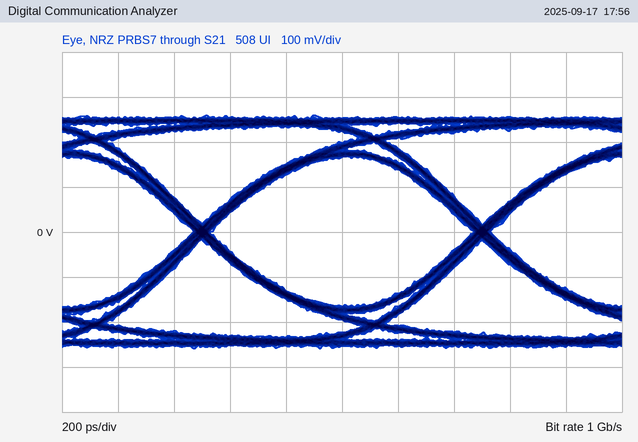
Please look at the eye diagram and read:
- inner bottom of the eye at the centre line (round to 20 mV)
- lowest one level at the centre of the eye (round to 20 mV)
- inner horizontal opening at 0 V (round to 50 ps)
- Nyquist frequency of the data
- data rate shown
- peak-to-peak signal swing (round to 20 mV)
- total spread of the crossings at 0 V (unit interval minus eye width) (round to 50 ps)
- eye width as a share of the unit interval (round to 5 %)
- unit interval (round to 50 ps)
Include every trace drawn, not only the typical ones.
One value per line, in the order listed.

-160 mV
160 mV
950 ps
500 MHz
1 Gb/s
520 mV
50 ps
95 %
1.00 ns
